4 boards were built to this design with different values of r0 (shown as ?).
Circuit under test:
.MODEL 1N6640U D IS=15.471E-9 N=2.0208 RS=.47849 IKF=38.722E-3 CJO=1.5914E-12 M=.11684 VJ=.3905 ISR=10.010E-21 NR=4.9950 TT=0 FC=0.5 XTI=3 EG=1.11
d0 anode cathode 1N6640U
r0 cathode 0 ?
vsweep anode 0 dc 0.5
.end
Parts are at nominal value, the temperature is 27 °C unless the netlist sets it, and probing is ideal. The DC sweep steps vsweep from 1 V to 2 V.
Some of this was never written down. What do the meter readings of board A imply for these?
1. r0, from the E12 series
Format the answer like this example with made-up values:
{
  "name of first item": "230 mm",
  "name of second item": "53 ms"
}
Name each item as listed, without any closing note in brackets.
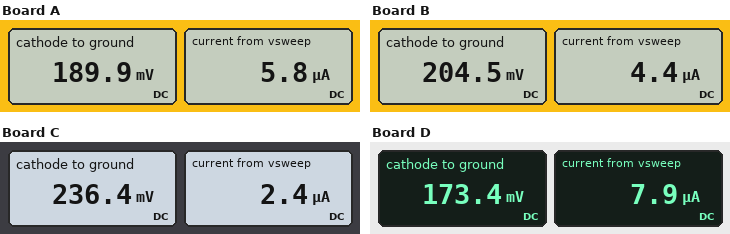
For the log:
{
  "r0, from the E12 series": "33 kΩ"
}
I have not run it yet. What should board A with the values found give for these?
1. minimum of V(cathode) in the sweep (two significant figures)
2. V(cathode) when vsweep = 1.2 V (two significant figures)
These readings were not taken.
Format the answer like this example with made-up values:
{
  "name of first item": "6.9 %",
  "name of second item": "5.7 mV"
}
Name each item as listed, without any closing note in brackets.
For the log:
{
  "minimum of V(cathode) in the sweep": "630 mV",
  "V(cathode) when vsweep = 1.2 V": "810 mV"
}
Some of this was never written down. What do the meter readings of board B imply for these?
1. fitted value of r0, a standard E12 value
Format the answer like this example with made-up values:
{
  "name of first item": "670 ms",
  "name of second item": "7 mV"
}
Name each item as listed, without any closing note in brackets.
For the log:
{
  "fitted value of r0, a standard E12 value": "47 kΩ"
}
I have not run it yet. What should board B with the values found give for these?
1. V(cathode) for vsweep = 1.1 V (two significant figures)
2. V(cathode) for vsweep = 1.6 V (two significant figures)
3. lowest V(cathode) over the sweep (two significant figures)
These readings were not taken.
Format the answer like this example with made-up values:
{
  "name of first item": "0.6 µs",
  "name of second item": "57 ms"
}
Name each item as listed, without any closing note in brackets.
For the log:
{
  "V(cathode) for vsweep = 1.1 V": "740 mV",
  "V(cathode) for vsweep = 1.6 V": "1.2 V",
  "lowest V(cathode) over the sweep": "640 mV"
}
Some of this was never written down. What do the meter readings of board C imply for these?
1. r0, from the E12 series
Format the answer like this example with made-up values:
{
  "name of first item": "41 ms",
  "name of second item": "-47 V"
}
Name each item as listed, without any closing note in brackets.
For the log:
{
  "r0, from the E12 series": "100 kΩ"
}
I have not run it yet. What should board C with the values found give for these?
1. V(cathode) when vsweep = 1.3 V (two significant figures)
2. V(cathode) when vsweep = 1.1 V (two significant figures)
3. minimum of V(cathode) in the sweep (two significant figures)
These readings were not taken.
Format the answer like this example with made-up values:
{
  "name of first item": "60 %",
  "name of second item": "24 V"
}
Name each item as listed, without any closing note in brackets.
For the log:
{
  "V(cathode) when vsweep = 1.3 V": "960 mV",
  "V(cathode) when vsweep = 1.1 V": "770 mV",
  "minimum of V(cathode) in the sweep": "680 mV"
}
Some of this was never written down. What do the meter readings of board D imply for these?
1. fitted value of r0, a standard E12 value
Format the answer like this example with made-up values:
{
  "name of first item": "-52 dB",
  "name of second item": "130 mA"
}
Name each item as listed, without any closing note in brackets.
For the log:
{
  "fitted value of r0, a standard E12 value": "22 kΩ"
}
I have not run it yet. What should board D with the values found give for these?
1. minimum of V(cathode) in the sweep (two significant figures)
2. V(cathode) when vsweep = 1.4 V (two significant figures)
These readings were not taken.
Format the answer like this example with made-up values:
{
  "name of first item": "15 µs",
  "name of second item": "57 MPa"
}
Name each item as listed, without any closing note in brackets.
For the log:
{
  "minimum of V(cathode) in the sweep": "610 mV",
  "V(cathode) when vsweep = 1.4 V": "980 mV"
}
